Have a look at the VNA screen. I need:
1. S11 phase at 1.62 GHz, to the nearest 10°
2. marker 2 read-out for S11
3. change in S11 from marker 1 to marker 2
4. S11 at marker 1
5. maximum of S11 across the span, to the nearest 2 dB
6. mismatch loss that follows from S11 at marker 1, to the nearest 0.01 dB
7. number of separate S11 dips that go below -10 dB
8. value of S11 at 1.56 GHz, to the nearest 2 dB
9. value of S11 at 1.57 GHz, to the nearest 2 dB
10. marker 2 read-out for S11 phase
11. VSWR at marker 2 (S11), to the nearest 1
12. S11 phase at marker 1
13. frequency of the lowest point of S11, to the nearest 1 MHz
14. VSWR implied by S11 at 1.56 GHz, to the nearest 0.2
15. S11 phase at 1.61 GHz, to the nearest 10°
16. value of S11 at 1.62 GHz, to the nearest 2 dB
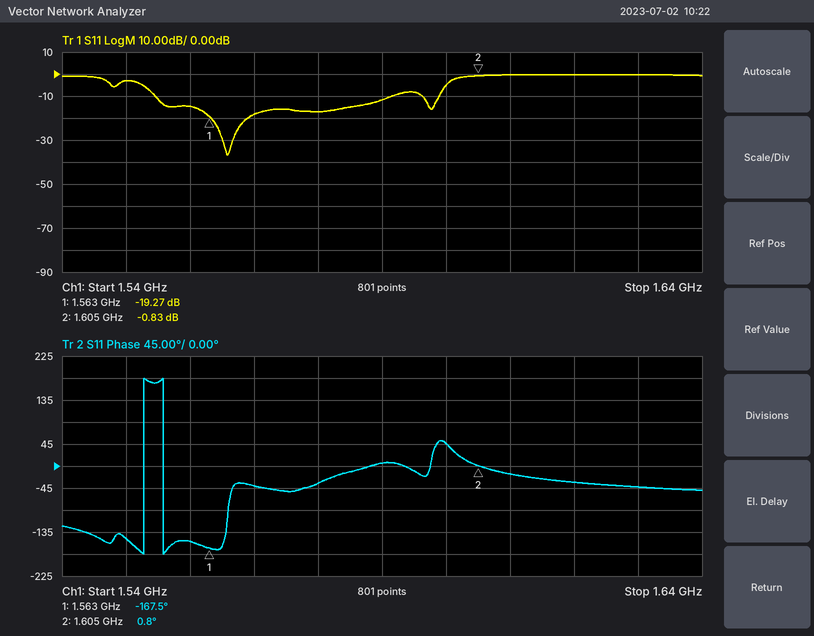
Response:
-30°
-0.83 dB
18.44 dB
-19.27 dB
0 dB
0.05 dB
2
-14 dB
-18 dB
0.8°
21
-167.5°
1.566 GHz
1.4
-20°
0 dB
